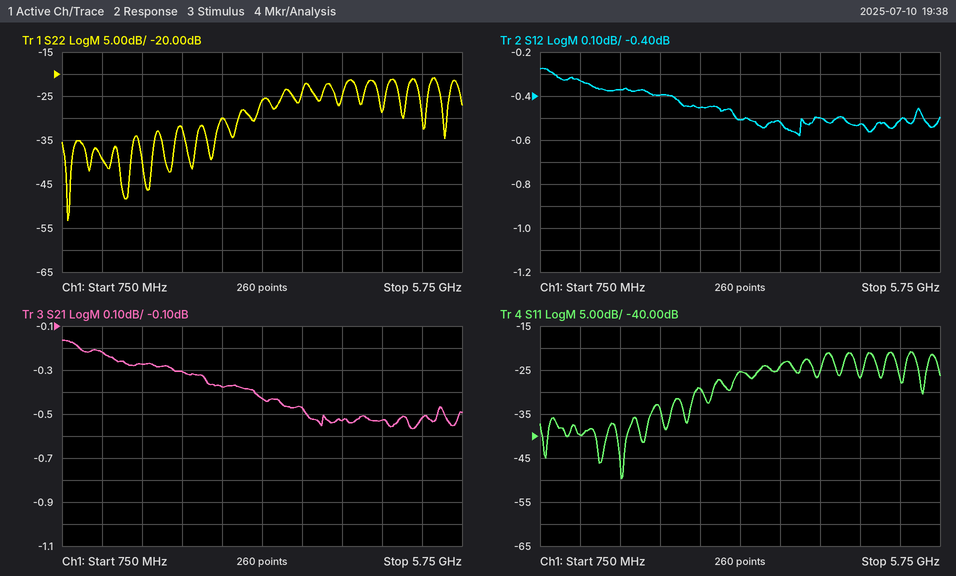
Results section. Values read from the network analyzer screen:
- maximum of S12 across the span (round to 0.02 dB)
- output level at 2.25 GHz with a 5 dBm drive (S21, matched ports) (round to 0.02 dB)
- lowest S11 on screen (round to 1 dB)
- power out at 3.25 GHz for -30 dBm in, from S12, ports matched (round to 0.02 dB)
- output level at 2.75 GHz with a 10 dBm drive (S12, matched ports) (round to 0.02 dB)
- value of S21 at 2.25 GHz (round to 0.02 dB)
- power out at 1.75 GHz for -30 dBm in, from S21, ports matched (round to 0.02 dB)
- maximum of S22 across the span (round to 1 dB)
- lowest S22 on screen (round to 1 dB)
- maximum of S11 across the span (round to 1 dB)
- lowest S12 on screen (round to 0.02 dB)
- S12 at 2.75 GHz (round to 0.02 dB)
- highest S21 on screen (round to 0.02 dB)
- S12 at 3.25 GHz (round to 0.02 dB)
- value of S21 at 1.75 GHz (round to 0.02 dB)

-0.28 dB
4.70 dBm
-50 dB
-30.50 dBm
9.54 dBm
-0.30 dB
-30.28 dBm
-21 dB
-53 dB
-21 dB
-0.58 dB
-0.46 dB
-0.16 dB
-0.50 dB
-0.28 dB
